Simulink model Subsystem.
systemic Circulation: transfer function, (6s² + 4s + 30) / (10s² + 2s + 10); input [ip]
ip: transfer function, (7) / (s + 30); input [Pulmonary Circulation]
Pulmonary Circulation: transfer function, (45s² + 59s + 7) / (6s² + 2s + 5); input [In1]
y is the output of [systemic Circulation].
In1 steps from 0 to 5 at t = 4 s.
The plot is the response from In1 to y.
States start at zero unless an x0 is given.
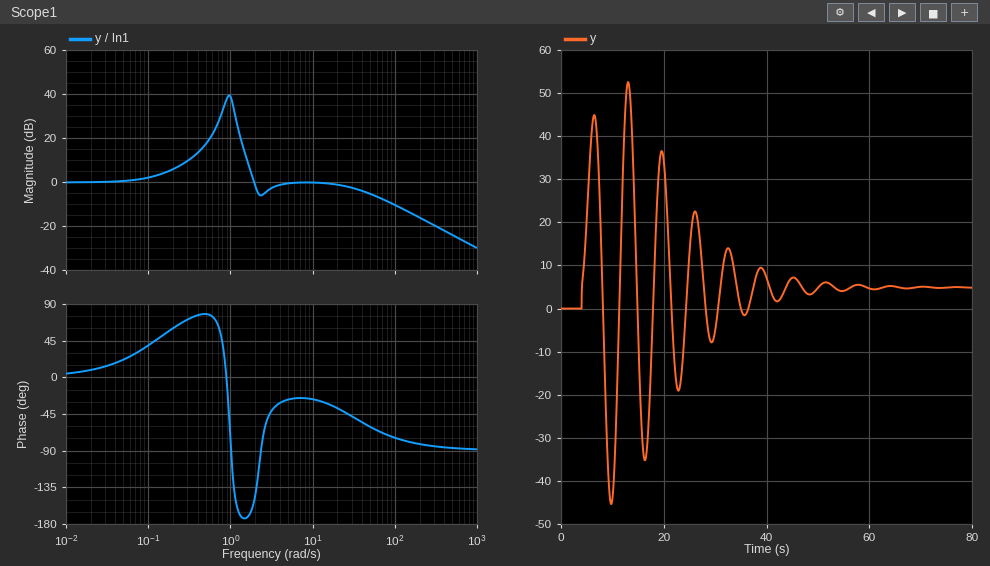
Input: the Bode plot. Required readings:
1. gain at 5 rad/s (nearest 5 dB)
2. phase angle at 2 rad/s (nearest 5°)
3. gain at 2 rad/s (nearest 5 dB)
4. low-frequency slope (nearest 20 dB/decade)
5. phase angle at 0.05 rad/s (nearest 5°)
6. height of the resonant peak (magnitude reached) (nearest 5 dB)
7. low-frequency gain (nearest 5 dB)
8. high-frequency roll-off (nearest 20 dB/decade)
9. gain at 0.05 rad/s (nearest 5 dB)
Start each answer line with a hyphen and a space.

- 0 dB
- -145°
- 0 dB
- 0 dB/decade
- 20°
- 40 dB
- 0 dB
- -20 dB/decade
- 0 dB
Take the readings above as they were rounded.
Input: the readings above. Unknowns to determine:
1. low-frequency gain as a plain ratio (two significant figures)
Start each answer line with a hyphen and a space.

- 1.0
